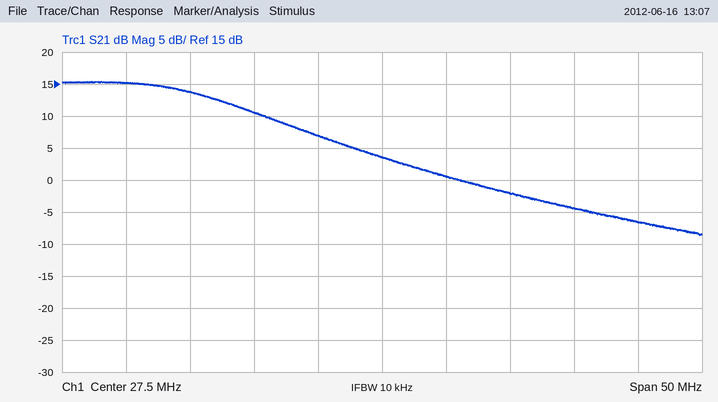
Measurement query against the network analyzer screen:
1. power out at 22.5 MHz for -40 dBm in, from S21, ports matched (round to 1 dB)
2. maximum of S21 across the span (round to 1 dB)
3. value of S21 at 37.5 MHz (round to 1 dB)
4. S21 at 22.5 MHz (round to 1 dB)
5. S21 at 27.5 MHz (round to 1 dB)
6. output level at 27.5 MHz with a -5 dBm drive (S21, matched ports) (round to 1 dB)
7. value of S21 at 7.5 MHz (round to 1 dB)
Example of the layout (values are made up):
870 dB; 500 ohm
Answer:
-33 dBm; 15 dB; -2 dB; 7 dB; 4 dB; -1 dBm; 15 dB
